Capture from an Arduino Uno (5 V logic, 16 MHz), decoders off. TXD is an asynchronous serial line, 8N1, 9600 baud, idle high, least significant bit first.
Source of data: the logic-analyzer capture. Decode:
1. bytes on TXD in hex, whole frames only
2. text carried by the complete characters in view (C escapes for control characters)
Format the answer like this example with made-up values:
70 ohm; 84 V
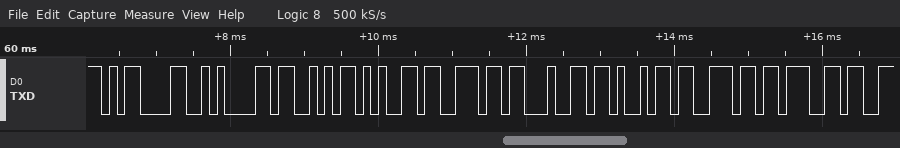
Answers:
0x0D 0x0A 0x53 0x65 0x6E 0x64 0x69 0x6E 0x67; "\r\nSending"
